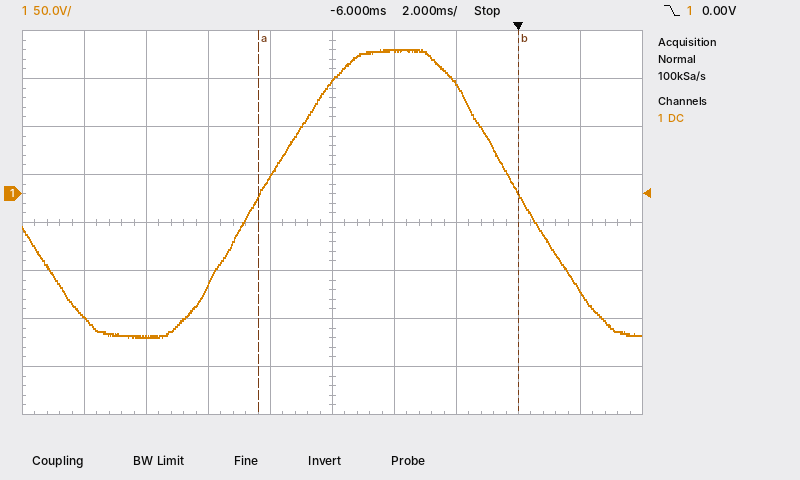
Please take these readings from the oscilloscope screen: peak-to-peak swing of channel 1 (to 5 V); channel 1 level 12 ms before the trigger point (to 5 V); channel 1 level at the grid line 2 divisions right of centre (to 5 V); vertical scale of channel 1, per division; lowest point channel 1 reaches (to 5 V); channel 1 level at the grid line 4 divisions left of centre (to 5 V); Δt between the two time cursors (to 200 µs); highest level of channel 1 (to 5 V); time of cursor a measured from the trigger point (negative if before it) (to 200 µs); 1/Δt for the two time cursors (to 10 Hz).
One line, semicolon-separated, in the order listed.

300 V; -150 V; 115 V; 50 V; -150 V; -130 V; 8.4 ms; 150 V; -8.4 ms; 120 Hz
